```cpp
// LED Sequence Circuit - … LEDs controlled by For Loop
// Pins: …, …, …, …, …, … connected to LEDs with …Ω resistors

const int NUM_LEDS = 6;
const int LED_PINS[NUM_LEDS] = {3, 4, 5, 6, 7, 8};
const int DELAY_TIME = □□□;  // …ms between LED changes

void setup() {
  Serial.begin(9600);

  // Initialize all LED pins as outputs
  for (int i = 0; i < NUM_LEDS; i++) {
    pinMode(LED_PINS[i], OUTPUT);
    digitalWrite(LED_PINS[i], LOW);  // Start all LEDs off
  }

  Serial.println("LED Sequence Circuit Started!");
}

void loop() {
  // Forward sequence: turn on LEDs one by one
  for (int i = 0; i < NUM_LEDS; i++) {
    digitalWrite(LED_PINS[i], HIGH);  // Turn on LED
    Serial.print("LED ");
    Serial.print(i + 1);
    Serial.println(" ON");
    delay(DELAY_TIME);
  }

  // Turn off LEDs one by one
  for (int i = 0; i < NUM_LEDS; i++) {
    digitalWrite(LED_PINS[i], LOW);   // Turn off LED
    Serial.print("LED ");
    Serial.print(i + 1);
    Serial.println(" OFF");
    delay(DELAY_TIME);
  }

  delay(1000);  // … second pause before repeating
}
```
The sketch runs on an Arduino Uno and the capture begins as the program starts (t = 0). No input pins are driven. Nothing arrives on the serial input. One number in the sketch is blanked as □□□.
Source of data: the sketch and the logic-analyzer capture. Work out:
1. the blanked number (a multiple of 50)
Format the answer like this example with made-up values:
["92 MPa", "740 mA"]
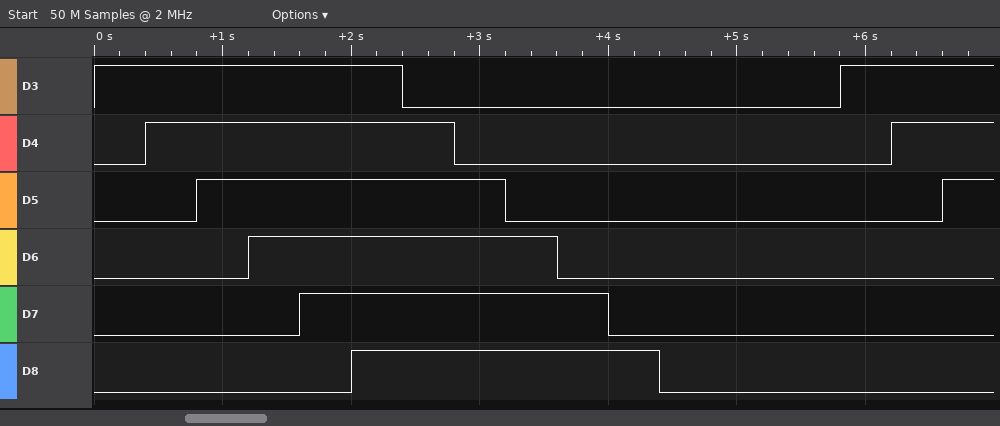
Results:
["400"]
